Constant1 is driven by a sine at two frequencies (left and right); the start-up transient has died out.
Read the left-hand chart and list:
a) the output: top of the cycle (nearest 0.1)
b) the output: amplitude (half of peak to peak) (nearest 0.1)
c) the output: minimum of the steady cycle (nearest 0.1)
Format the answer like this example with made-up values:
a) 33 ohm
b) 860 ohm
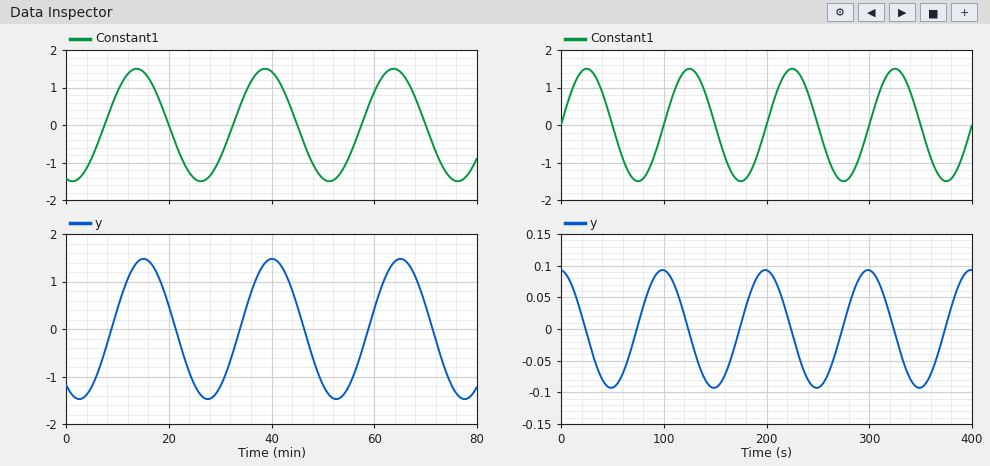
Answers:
a) 1.5
b) 1.5
c) -1.5
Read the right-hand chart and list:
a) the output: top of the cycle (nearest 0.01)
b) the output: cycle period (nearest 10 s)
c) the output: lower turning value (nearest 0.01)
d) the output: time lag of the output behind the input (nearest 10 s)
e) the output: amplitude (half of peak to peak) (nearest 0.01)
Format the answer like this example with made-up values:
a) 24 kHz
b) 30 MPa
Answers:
a) 0.09
b) 100 s
c) -0.09
d) 70 s
e) 0.09
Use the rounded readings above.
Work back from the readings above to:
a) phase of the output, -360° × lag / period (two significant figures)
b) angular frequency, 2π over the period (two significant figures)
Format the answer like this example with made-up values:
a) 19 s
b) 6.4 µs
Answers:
a) -250°
b) 0.063 rad/s
